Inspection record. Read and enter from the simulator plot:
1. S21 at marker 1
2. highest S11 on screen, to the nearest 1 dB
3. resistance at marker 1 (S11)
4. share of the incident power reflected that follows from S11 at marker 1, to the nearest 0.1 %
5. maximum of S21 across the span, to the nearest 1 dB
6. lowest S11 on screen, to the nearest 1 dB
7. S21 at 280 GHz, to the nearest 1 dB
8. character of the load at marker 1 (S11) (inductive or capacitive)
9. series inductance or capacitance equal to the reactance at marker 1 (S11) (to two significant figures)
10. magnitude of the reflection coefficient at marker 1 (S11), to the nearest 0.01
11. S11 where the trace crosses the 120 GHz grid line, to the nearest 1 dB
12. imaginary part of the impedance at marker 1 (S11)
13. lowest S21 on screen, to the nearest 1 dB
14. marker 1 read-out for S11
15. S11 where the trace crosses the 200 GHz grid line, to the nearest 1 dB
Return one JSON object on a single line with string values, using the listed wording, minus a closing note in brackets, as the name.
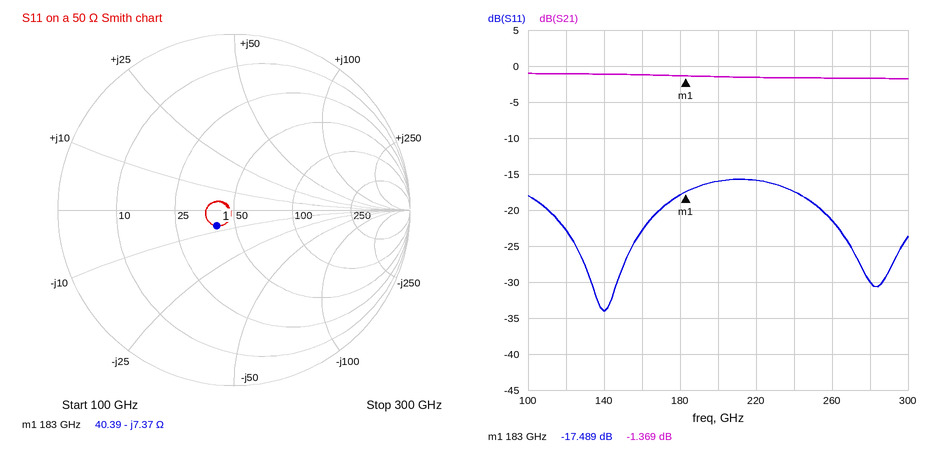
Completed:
{"S21 at marker 1": "-1.369 dB", "highest S11 on screen, to the nearest 1 dB": "-16 dB", "resistance at marker 1": "40.39 Ω", "share of the incident power reflected that follows from S11 at marker 1, to the nearest 0.1 %": "1.8 %", "maximum of S21 across the span, to the nearest 1 dB": "-1 dB", "lowest S11 on screen, to the nearest 1 dB": "-34 dB", "S21 at 280 GHz, to the nearest 1 dB": "-2 dB", "character of the load at marker 1 (S11)": "capacitive", "series inductance or capacitance equal to the reactance at marker 1 (S11)": "120 fF", "magnitude of the reflection coefficient at marker 1 (S11), to the nearest 0.01": "0.13", "S11 where the trace crosses the 120 GHz grid line, to the nearest 1 dB": "-23 dB", "imaginary part of the impedance at marker 1": "-7.37 Ω", "lowest S21 on screen, to the nearest 1 dB": "-2 dB", "marker 1 read-out for S11": "-17.489 dB", "S11 where the trace crosses the 200 GHz grid line, to the nearest 1 dB": "-16 dB"}
